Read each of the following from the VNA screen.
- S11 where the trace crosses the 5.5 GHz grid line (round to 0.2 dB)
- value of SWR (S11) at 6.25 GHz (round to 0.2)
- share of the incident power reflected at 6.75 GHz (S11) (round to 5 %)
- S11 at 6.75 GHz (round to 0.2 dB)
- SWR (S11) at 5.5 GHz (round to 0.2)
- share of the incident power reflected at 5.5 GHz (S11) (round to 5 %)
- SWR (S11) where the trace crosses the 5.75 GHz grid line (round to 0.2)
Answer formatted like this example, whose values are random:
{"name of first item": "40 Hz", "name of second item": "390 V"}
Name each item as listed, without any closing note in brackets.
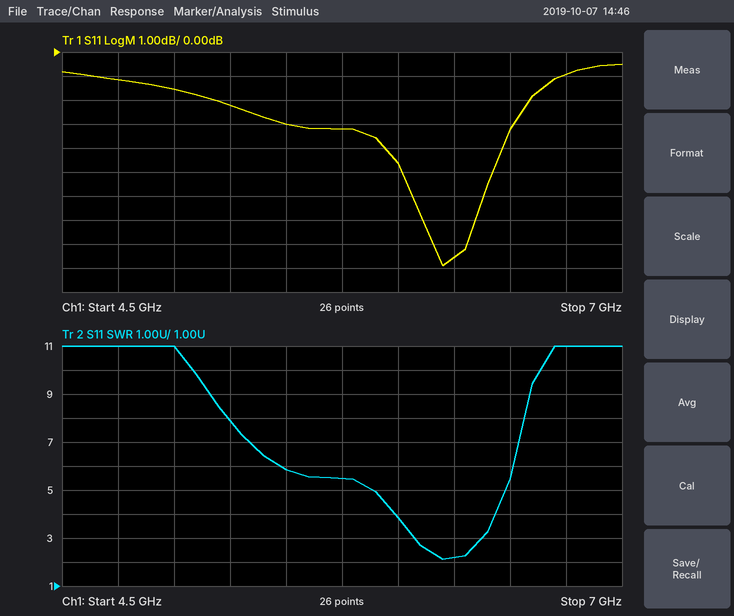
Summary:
{"S11 where the trace crosses the 5.5 GHz grid line": "-3.0 dB", "value of SWR (S11) at 6.25 GHz": "2.2", "share of the incident power reflected at 6.75 GHz (S11)": "80 %", "S11 at 6.75 GHz": "-1.0 dB", "SWR (S11) at 5.5 GHz": "5.8", "share of the incident power reflected at 5.5 GHz (S11)": "50 %", "SWR (S11) where the trace crosses the 5.75 GHz grid line": "5.4"}
